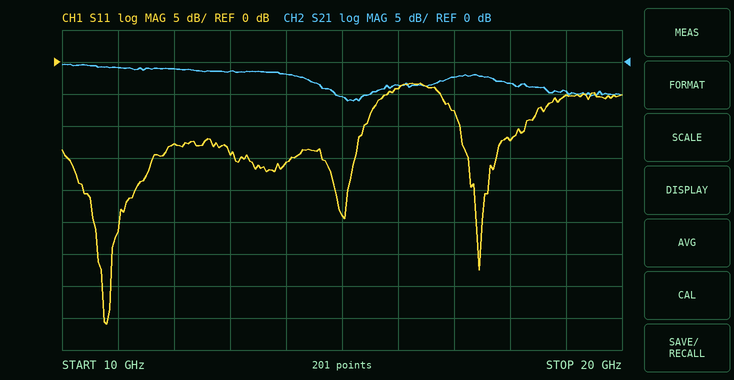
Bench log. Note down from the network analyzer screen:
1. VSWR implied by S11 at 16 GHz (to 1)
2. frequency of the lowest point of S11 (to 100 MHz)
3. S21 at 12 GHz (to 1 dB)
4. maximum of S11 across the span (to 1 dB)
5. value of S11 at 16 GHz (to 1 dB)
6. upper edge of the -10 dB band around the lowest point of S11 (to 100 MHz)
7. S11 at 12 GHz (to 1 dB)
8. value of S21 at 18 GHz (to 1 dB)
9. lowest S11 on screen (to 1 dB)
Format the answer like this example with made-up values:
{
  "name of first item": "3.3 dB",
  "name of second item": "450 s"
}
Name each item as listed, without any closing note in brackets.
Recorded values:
{
  "VSWR implied by S11 at 16 GHz": "4",
  "frequency of the lowest point of S11": "10.8 GHz",
  "S21 at 12 GHz": "-1 dB",
  "maximum of S11 across the span": "-3 dB",
  "value of S11 at 16 GHz": "-4 dB",
  "upper edge of the -10 dB band around the lowest point of S11": "15.4 GHz",
  "S11 at 12 GHz": "-13 dB",
  "value of S21 at 18 GHz": "-3 dB",
  "lowest S11 on screen": "-41 dB"
}
